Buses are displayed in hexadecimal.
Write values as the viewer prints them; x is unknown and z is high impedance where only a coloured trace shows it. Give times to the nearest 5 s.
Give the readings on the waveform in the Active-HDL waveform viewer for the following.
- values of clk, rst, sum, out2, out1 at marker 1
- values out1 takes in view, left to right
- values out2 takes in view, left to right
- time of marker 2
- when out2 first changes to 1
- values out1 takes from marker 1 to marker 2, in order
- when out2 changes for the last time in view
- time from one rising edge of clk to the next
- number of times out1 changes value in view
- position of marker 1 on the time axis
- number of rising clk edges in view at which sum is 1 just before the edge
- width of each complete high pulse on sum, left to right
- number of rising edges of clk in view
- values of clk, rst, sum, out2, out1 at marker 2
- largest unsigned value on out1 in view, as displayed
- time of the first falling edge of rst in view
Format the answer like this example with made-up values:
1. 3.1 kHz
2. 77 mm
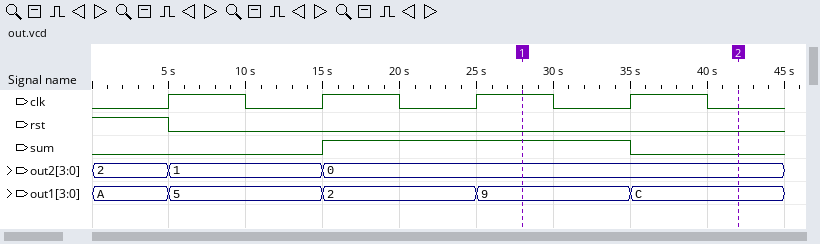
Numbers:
1. clk=1, rst=0, sum=1, out2=0, out1=9
2. A, 5, 2, 9, C
3. 2, 1, 0
4. 40 s
5. 5 s
6. 9, C
7. 15 s
8. 10 s
9. 4
10. 30 s
11. 2
12. 20 s
13. 4
14. clk=0, rst=0, sum=0, out2=0, out1=C
15. C
16. 5 s
